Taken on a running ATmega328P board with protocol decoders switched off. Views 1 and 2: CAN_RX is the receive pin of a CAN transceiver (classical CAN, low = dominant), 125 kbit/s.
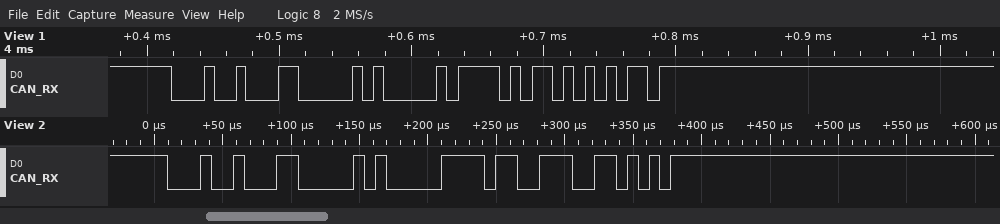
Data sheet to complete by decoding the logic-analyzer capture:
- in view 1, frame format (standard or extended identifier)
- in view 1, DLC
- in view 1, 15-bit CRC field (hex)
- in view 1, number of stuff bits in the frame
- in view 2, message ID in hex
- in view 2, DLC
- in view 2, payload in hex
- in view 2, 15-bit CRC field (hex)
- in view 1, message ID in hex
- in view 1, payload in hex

standard
1
0x6B55
2
0x123
1
07
0x339A
0x123
03
